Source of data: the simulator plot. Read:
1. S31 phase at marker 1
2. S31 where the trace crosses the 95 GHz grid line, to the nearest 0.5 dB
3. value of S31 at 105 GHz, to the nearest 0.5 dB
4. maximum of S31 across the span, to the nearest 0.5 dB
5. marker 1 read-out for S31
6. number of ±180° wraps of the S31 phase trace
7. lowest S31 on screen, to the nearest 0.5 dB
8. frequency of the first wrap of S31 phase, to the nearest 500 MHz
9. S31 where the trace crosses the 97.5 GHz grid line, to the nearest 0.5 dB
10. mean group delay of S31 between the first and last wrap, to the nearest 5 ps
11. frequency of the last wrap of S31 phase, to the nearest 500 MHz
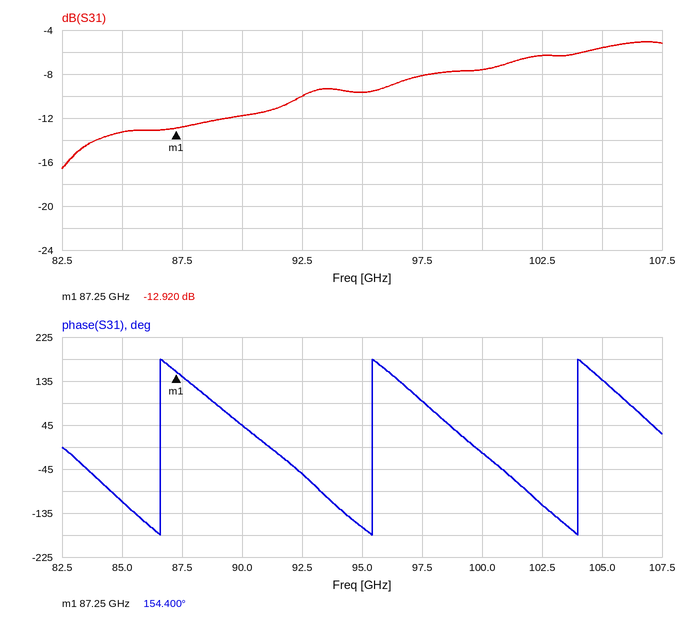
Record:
154.400°
-9.5 dB
-5.5 dB
-5.0 dB
-12.920 dB
3
-16.5 dB
86.5 GHz
-8.0 dB
115 ps
104.0 GHz
